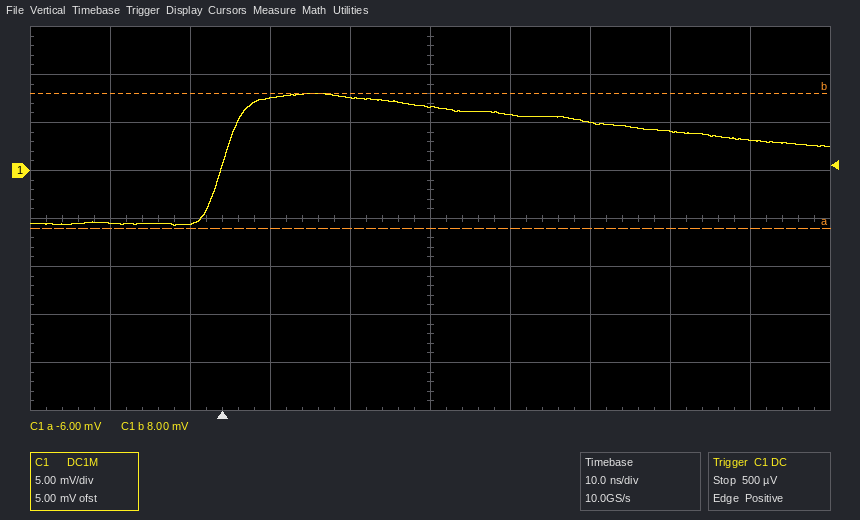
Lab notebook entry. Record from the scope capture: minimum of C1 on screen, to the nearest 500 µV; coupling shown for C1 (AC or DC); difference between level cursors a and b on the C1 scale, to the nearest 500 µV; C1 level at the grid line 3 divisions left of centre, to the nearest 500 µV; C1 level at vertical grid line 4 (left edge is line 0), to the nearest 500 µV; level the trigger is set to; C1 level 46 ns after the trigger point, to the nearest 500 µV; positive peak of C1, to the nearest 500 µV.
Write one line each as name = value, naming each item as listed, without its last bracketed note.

minimum of C1 on screen, to the nearest 500 µV = -5.5 mV
coupling shown for C1 = DC
difference between level cursors a and b on the C1 scale, to the nearest 500 µV = 14.0 mV
C1 level at the grid line 3 divisions left of centre, to the nearest 500 µV = -5.5 mV
C1 level at vertical grid line 4 (left edge is line 0), to the nearest 500 µV = 7.5 mV
level the trigger is set to = 500 µV
C1 level 46 ns after the trigger point, to the nearest 500 µV = 5.0 mV
positive peak of C1, to the nearest 500 µV = 8.0 mV
